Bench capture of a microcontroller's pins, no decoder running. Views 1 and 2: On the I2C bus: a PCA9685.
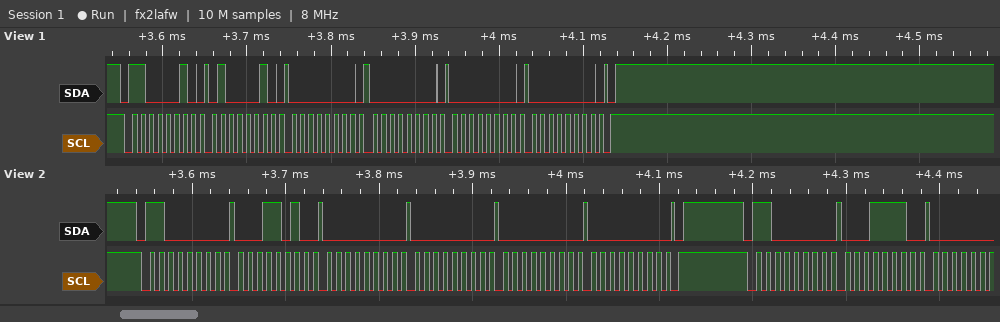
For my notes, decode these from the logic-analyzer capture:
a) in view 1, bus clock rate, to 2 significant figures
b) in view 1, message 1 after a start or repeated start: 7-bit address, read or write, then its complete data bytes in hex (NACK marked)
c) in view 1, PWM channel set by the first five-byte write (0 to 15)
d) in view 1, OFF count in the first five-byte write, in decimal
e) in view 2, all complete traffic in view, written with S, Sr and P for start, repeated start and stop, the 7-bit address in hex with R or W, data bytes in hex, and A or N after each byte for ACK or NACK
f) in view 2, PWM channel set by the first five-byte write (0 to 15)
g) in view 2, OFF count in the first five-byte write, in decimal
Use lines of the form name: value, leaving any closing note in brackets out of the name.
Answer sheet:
in view 1, bus clock rate, to 2 significant figures: 100 kHz
in view 1, message 1 after a start or repeated start: 7-bit address, read or write, then its complete data bytes in hex: 0x61 write: 42 00 00 00 00
in view 1, PWM channel set by the first five-byte write: 15
in view 1, OFF count in the first five-byte write, in decimal: 0
in view 2, all complete traffic in view, written with S, Sr and P for start, repeated start and stop, the 7-bit address in hex with R or W, data bytes in hex, and A or N after each byte for ACK or NACK: S 60W A 1A A 00 A 00 A 00 A 00 A P S 60W A 1E A
in view 2, PWM channel set by the first five-byte write: 5
in view 2, OFF count in the first five-byte write, in decimal: 0
